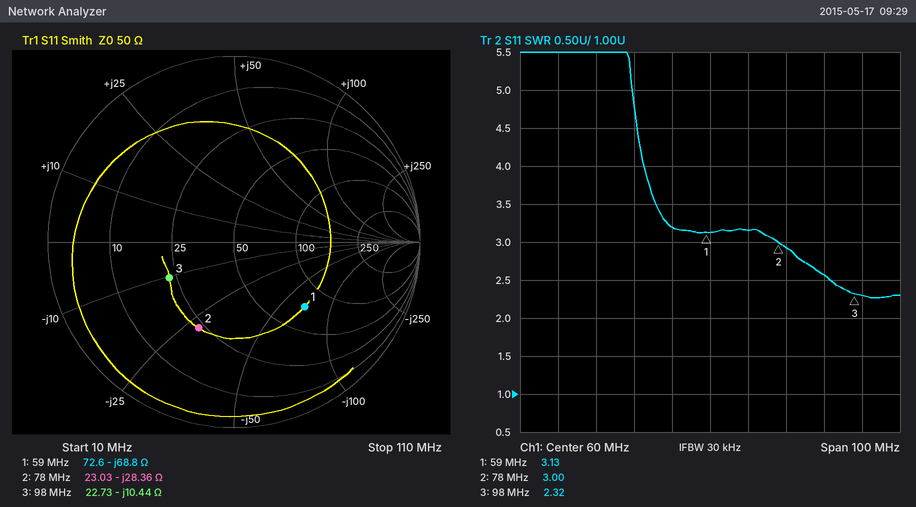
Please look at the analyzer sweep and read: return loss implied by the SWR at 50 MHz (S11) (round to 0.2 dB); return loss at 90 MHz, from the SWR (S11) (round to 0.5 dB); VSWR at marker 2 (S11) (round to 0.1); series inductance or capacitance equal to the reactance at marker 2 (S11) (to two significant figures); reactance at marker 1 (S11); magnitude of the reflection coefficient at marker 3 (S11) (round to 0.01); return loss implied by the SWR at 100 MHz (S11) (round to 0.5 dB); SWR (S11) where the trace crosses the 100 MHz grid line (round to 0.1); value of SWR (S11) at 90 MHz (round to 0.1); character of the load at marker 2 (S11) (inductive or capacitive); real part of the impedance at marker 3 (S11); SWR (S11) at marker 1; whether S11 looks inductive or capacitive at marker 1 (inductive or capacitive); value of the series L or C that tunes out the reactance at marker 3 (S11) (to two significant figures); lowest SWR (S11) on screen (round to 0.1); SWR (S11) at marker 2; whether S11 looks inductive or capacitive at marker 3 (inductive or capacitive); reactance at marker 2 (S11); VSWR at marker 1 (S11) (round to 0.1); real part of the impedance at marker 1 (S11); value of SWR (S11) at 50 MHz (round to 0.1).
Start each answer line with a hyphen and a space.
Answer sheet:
- 5.6 dB
- 7.0 dB
- 3.0
- 72 pF
- -68.8 Ω
- 0.40
- 8.0 dB
- 2.3
- 2.6
- capacitive
- 22.73 Ω
- 3.13
- capacitive
- 17 nH
- 2.3
- 3.00
- capacitive
- -28.36 Ω
- 3.1
- 72.6 Ω
- 3.2
